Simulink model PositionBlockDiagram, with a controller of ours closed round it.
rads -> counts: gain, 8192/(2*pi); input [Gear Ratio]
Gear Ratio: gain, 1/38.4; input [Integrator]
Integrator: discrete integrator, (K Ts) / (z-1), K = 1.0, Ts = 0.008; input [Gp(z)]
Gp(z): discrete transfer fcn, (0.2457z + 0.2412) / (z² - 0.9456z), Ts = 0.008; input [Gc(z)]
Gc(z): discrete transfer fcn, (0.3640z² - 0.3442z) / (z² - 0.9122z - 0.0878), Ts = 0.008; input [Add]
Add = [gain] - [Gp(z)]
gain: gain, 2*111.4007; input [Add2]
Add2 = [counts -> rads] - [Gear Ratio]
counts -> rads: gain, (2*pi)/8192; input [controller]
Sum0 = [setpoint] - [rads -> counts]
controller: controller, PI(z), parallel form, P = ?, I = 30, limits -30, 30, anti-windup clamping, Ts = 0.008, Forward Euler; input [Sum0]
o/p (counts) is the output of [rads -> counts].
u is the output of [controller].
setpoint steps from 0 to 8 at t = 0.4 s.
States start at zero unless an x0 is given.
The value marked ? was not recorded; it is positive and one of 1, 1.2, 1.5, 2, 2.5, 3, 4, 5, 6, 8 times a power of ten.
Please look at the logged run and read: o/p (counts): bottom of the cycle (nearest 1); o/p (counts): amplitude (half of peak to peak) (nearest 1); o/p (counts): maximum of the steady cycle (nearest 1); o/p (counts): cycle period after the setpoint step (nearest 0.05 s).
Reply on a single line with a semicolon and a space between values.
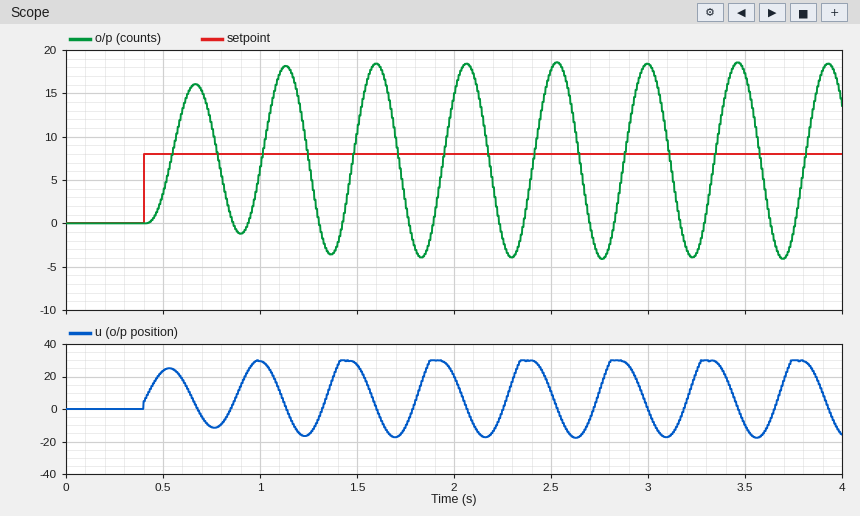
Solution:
-4; 11; 19; 0.45 s
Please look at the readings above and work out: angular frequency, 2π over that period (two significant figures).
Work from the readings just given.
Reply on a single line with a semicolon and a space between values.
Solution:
14 rad/s
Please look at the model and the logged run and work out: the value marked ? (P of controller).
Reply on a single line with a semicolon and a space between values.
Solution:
0.6
